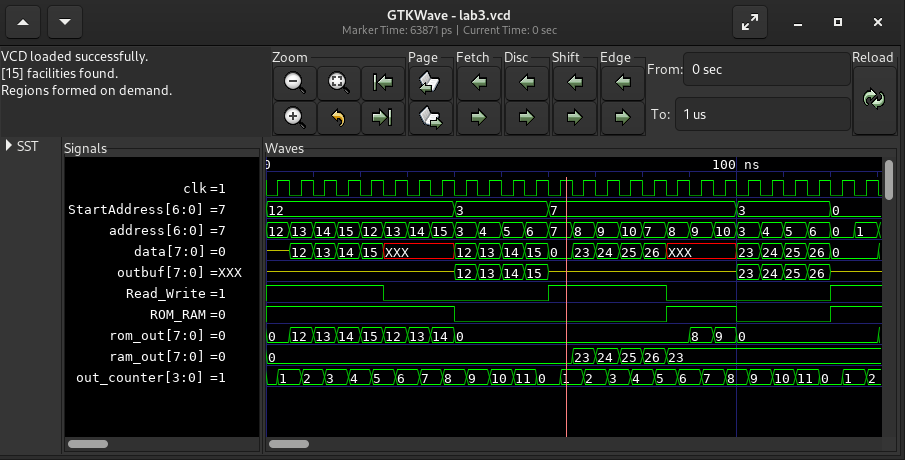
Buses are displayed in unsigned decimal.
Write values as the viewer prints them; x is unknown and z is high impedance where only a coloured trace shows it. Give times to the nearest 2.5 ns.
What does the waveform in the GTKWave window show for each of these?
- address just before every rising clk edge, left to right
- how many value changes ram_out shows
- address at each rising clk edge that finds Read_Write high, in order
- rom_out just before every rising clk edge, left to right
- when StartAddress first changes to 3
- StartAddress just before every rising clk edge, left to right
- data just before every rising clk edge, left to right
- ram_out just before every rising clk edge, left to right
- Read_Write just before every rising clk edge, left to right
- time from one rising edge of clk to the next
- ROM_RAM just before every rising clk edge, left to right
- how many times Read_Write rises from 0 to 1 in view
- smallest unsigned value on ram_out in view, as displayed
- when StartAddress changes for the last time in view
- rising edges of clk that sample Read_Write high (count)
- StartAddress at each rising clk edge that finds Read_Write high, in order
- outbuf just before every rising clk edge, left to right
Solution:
12, 13, 14, 15, 12, 13, 14, 15, 3, 4, 5, 6, 7, 8, 9, 10, 7, 8, 9, 10, 3, 4, 5, 6, 0, 1
5
12, 13, 14, 15, 12, 7, 8, 9, 10, 7, 0, 1
0, 12, 13, 14, 15, 12, 13, 14, 0, 0, 0, 0, 0, 0, 0, 0, 0, 0, 8, 9, 0, 0, 0, 0, 0, 0
40 ns
12, 12, 12, 12, 12, 12, 12, 12, 3, 3, 3, 3, 7, 7, 7, 7, 7, 7, 7, 7, 3, 3, 3, 3, 0, 0
z, 12, 13, 14, 15, XXX, XXX, XXX, 12, 13, 14, 15, 0, 23, 24, 25, 26, XXX, XXX, XXX, 23, 24, 25, 26, 0, 0
0, 0, 0, 0, 0, 0, 0, 0, 0, 0, 0, 0, 0, 23, 24, 25, 26, 23, 23, 23, 23, 23, 23, 23, 23, 23
1 1 1 1 1 0 0 0 0 0 0 0 1 1 1 1 1 0 0 0 0 0 0 0 1 1
5 ns
1 1 1 1 1 1 1 1 0 0 0 0 0 0 0 0 0 1 1 1 0 0 0 0 1 1
2
0
120 ns
12
12, 12, 12, 12, 12, 7, 7, 7, 7, 7, 0, 0
z, z, z, z, z, z, z, z, 12, 13, 14, 15, z, z, z, z, z, z, z, z, 23, 24, 25, 26, z, z
